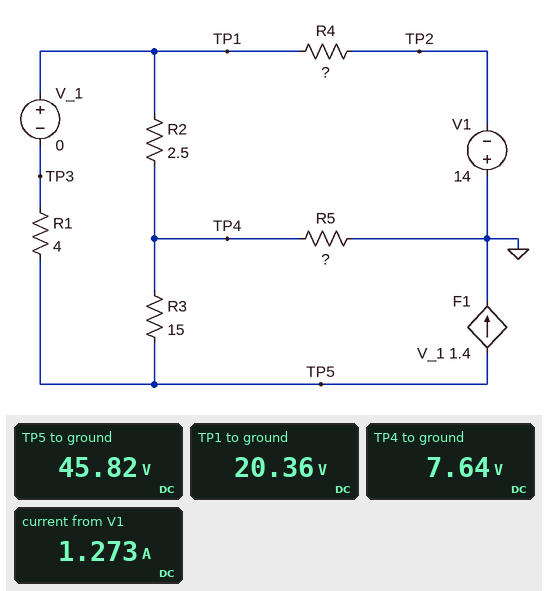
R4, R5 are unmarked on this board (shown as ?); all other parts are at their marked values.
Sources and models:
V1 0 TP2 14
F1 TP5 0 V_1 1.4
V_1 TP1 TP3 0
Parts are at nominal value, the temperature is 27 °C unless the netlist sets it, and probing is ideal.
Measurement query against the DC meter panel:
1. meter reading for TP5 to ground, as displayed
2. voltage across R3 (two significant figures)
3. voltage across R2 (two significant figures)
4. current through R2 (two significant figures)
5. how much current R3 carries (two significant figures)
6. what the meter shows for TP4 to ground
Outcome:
45.82 V
38 V
13 V
5.1 A
2.5 A
7.64 V
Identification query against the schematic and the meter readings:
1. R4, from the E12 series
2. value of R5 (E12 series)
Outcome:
27 Ω
1 Ω
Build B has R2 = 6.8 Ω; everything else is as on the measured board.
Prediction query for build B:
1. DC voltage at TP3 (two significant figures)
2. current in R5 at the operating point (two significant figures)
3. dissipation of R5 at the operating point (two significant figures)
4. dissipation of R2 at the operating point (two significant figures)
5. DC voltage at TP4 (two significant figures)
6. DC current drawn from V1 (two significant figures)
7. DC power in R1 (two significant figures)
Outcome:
2.3 V
590 mA
350 mW
430 mW
590 mV
600 mA
2.9 W
